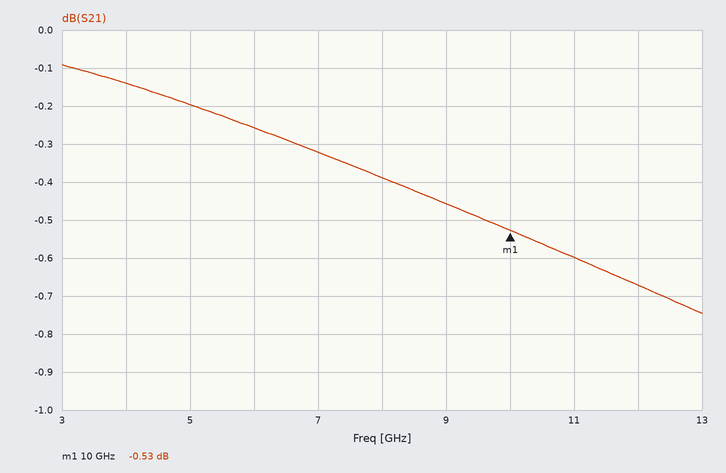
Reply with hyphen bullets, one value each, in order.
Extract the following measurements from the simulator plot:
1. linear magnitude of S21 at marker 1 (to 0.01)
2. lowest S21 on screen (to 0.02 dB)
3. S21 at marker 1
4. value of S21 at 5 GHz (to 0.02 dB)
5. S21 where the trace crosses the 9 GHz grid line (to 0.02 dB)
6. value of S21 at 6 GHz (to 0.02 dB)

- 0.94
- -0.74 dB
- -0.53 dB
- -0.20 dB
- -0.46 dB
- -0.26 dB
